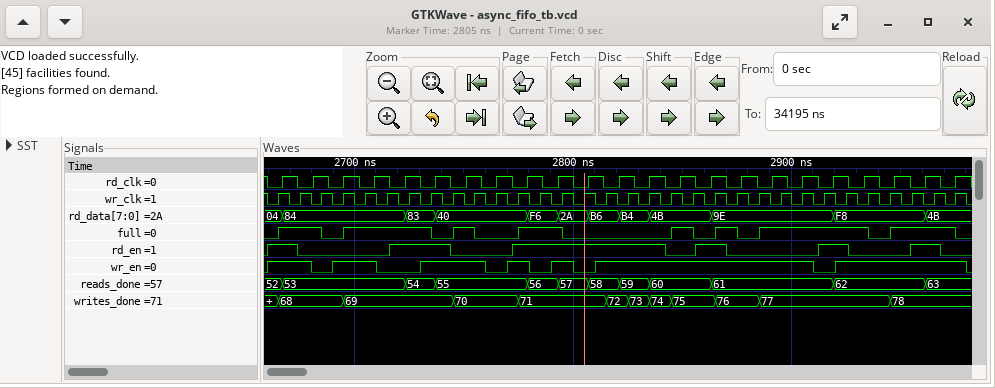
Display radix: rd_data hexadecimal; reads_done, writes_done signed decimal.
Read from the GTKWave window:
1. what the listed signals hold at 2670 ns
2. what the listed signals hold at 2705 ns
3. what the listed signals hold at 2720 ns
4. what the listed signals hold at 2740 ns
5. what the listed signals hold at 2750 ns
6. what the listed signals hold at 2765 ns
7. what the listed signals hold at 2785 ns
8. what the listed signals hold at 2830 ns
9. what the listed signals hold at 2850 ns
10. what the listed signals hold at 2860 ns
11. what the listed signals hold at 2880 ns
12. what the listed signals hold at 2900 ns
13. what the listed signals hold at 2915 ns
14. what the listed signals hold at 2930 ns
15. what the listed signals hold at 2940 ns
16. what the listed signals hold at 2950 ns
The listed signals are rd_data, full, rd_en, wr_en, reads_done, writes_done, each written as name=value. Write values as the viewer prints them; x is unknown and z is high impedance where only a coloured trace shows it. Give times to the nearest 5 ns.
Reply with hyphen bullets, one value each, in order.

- rd_data=84, full=1, rd_en=1, wr_en=1, reads_done=53, writes_done=68
- rd_data=84, full=1, rd_en=0, wr_en=1, reads_done=53, writes_done=69
- rd_data=84, full=1, rd_en=1, wr_en=0, reads_done=53, writes_done=69
- rd_data=40, full=0, rd_en=1, wr_en=1, reads_done=55, writes_done=69
- rd_data=40, full=1, rd_en=0, wr_en=1, reads_done=55, writes_done=70
- rd_data=40, full=0, rd_en=0, wr_en=0, reads_done=55, writes_done=70
- rd_data=F6, full=1, rd_en=1, wr_en=0, reads_done=56, writes_done=71
- rd_data=B4, full=0, rd_en=1, wr_en=1, reads_done=59, writes_done=73
- rd_data=4B, full=1, rd_en=0, wr_en=1, reads_done=60, writes_done=75
- rd_data=4B, full=0, rd_en=1, wr_en=1, reads_done=60, writes_done=75
- rd_data=9E, full=0, rd_en=0, wr_en=1, reads_done=61, writes_done=76
- rd_data=9E, full=1, rd_en=0, wr_en=1, reads_done=61, writes_done=77
- rd_data=9E, full=1, rd_en=1, wr_en=0, reads_done=61, writes_done=77
- rd_data=F8, full=1, rd_en=0, wr_en=1, reads_done=62, writes_done=77
- rd_data=F8, full=0, rd_en=0, wr_en=1, reads_done=62, writes_done=77
- rd_data=F8, full=1, rd_en=0, wr_en=1, reads_done=62, writes_done=78
